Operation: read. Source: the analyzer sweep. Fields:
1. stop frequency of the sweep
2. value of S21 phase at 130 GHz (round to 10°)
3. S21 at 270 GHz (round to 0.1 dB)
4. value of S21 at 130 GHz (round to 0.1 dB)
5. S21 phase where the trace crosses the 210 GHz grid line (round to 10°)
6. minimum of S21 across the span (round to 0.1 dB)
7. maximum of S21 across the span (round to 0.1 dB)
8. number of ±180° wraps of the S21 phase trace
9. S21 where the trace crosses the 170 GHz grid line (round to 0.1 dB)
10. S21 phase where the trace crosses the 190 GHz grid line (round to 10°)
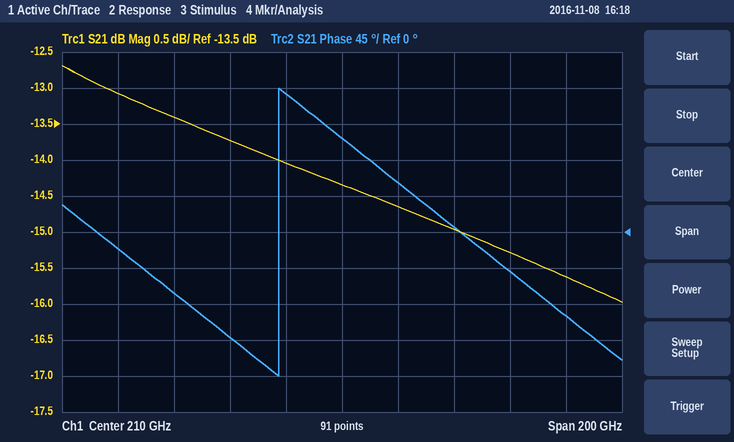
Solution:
310 GHz
-20°
-15.3 dB
-13.1 dB
120°
-16.0 dB
-12.7 dB
1
-13.7 dB
170°
